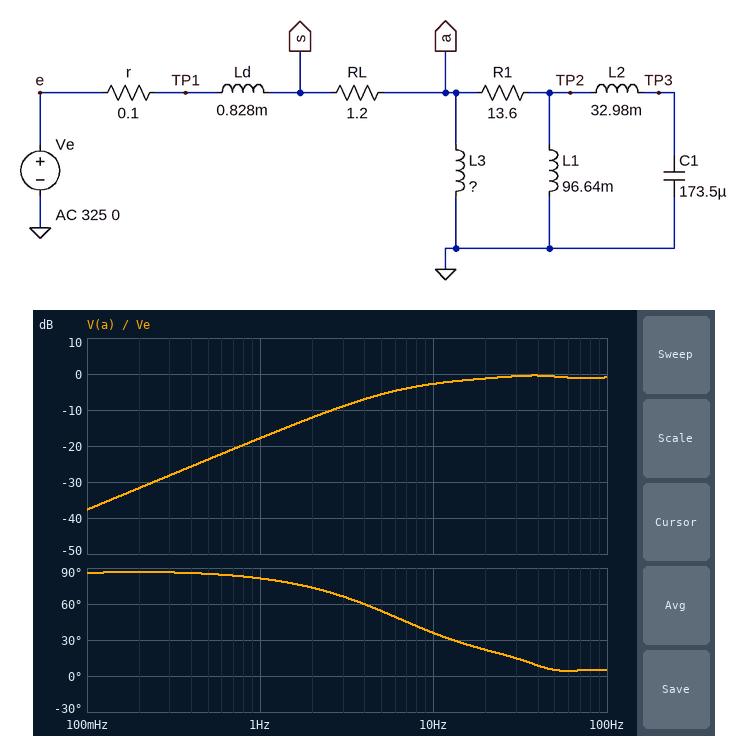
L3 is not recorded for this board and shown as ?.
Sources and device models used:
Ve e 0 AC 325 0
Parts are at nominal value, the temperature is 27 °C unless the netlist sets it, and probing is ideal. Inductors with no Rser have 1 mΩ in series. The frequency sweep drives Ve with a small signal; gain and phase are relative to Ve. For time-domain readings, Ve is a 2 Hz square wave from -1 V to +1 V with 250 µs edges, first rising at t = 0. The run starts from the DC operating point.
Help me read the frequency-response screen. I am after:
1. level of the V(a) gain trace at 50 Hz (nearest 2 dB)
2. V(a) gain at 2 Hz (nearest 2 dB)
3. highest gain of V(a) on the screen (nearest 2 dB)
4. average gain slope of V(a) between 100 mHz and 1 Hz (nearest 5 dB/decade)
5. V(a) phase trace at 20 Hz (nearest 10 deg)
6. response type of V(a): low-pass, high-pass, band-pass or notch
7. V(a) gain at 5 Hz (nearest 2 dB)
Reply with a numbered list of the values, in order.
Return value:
1. 0 dB
2. -12 dB
3. 0 dB
4. 20 dB/decade
5. 20 deg
6. high-pass
7. -6 dB
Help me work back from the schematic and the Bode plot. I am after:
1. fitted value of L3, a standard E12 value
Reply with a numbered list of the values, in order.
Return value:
1. 27 mH
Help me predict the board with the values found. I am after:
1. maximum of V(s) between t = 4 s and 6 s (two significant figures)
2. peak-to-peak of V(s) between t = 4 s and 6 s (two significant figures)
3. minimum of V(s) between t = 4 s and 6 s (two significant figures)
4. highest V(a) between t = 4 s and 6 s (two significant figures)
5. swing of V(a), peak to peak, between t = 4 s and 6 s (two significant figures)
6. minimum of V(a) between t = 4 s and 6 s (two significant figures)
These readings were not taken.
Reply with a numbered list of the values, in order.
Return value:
1. 1.0 V
2. 2.0 V
3. -1.0 V
4. 1.9 V
5. 3.7 V
6. -1.9 V
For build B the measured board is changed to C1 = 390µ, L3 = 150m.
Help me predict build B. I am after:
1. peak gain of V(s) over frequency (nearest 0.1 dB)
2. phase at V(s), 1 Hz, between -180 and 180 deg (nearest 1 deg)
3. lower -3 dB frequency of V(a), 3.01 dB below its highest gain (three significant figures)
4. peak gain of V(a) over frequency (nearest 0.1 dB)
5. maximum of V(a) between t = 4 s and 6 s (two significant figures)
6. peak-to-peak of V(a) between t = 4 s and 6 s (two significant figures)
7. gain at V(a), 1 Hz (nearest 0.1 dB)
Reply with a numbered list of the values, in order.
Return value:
1. 0 dB
2. 2 deg
3. 1.54 Hz
4. -0.1 dB
5. 1.7 V
6. 3.4 V
7. -5.0 dB
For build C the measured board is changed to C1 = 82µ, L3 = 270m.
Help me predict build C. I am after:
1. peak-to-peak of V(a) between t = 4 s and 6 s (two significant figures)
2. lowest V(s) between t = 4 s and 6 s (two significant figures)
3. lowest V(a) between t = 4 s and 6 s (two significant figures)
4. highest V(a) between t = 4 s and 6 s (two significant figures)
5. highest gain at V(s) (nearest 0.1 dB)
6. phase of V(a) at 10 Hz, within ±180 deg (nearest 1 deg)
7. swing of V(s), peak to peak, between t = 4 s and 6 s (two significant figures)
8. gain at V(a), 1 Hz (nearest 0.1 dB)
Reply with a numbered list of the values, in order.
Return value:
1. 2.9 V
2. -1.0 V
3. -1.5 V
4. 1.5 V
5. 0.1 dB
6. 6 deg
7. 2.1 V
8. -2.6 dB
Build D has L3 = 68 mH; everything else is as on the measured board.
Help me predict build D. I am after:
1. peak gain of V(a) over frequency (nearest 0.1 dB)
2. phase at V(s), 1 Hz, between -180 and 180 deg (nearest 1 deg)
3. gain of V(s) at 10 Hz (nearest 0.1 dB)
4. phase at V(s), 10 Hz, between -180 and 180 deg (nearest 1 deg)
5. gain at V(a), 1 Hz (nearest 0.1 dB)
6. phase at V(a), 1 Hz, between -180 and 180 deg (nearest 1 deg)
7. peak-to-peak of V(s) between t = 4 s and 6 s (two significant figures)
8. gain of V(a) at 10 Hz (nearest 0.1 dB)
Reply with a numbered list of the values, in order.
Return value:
1. -0.1 dB
2. 1 deg
3. -0.2 dB
4. 1 deg
5. -10.2 dB
6. 70 deg
7. 2.1 V
8. -1.2 dB
